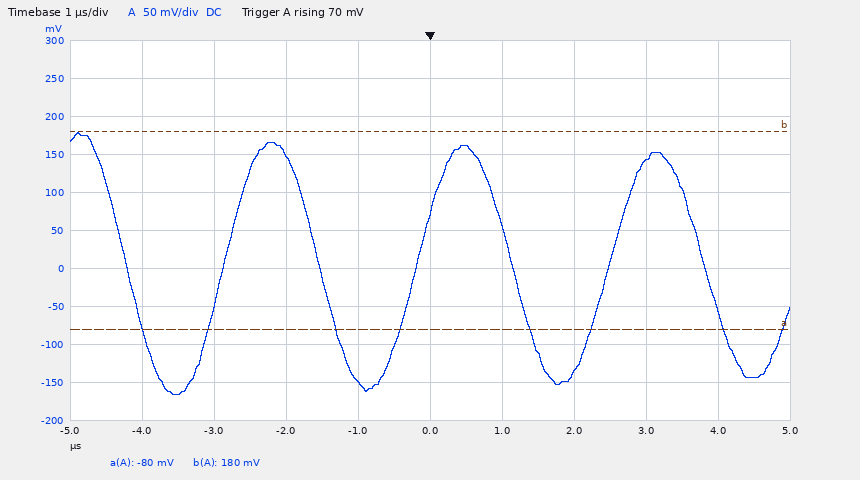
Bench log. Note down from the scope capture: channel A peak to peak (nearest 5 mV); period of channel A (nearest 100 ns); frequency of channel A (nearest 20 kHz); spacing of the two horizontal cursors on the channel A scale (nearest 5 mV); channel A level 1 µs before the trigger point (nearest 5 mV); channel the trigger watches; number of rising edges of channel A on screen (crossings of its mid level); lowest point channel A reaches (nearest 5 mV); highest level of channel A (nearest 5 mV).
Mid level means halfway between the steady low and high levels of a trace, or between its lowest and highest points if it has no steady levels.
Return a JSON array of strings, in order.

["345 mV", "2.7 µs", "380 kHz", "260 mV", "-150 mV", "channel A", "3", "-165 mV", "180 mV"]
